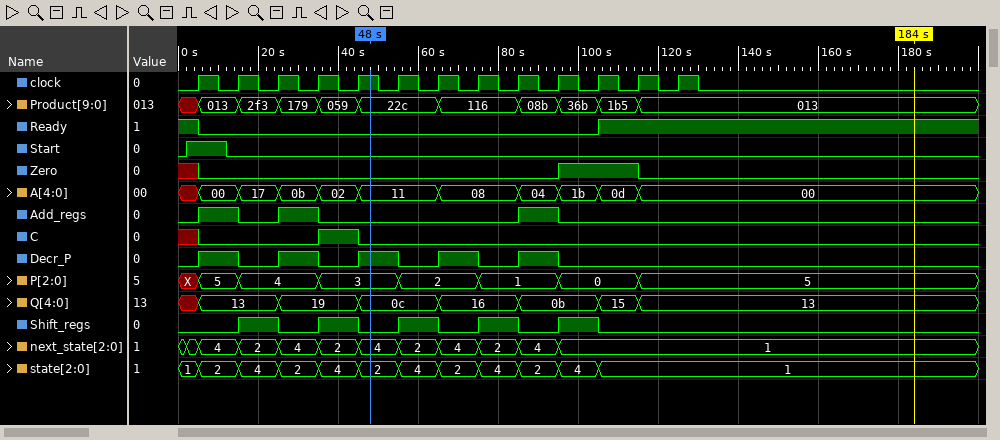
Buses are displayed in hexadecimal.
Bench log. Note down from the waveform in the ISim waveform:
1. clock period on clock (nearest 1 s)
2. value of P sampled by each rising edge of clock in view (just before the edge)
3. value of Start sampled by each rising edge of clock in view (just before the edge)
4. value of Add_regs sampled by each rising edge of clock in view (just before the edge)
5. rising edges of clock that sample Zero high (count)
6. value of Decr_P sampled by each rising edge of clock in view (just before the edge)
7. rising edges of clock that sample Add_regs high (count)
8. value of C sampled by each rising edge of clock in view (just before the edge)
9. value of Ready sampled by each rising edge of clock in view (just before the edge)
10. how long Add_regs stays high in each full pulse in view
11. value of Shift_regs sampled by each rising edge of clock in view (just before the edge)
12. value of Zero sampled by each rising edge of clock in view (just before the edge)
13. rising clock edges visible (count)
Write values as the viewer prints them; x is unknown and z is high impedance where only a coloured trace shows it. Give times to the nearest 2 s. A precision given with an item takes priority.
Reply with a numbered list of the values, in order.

1. 10 s
2. X, 5, 4, 4, 3, 3, 2, 2, 1, 1, 0, 0, 5
3. 1 0 0 0 0 0 0 0 0 0 0 0 0
4. 0 1 0 1 0 0 0 0 0 1 0 0 0
5. 2
6. 0 1 0 1 0 1 0 1 0 1 0 0 0
7. 3
8. x 0 0 0 1 0 0 0 0 0 0 0 0
9. 1 0 0 0 0 0 0 0 0 0 0 1 1
10. 10 s, 10 s, 10 s
11. 0 0 1 0 1 0 1 0 1 0 1 0 0
12. x 0 0 0 0 0 0 0 0 0 1 1 0
13. 13
